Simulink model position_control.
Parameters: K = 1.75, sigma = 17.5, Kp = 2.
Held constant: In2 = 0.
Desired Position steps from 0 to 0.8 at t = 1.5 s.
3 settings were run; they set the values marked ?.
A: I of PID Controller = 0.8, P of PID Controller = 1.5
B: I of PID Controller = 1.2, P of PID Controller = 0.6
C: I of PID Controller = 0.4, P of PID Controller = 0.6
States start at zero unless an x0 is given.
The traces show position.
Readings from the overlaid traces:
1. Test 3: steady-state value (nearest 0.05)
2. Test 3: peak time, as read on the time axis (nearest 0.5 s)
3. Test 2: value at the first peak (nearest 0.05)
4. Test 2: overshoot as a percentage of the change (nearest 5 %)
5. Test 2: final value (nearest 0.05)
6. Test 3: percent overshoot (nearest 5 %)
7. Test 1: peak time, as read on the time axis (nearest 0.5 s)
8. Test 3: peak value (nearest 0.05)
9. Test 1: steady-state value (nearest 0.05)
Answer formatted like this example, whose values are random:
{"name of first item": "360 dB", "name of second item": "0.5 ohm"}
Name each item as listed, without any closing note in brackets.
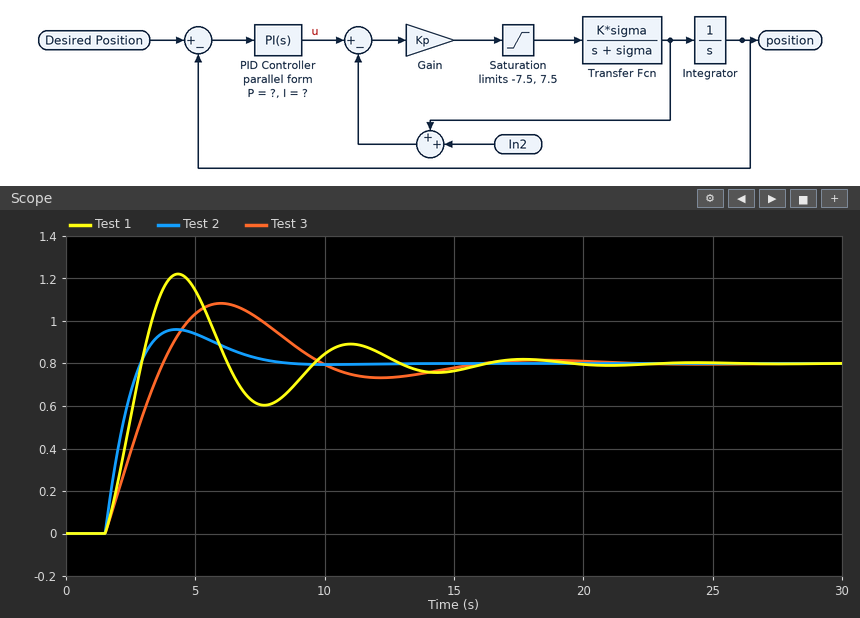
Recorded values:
{"Test 3: steady-state value": "0.80", "Test 3: peak time, as read on the time axis": "6.0 s", "Test 2: value at the first peak": "0.95", "Test 2: overshoot as a percentage of the change": "20 %", "Test 2: final value": "0.80", "Test 3: percent overshoot": "35 %", "Test 1: peak time, as read on the time axis": "4.5 s", "Test 3: peak value": "1.10", "Test 1: steady-state value": "0.80"}
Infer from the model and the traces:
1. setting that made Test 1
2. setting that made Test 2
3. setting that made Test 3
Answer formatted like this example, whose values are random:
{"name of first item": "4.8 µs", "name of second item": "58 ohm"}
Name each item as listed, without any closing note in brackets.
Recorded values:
{"setting that made Test 1": "B", "setting that made Test 2": "A", "setting that made Test 3": "C"}
